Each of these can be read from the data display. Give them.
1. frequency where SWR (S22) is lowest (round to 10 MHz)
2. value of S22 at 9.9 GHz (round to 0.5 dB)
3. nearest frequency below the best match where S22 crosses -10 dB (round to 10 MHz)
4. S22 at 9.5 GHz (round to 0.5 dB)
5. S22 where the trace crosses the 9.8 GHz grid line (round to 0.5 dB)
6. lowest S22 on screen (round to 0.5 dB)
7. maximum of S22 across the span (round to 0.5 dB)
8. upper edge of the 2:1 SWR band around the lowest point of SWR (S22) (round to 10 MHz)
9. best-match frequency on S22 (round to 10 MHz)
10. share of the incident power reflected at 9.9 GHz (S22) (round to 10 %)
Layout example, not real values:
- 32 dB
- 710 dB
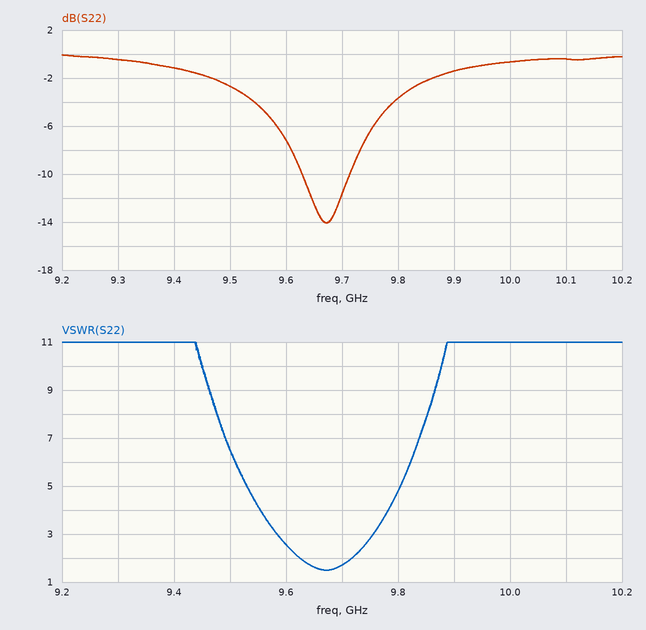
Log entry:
- 9.67 GHz
- -1.5 dB
- 9.63 GHz
- -2.5 dB
- -3.5 dB
- -14.0 dB
- 0.0 dB
- 9.72 GHz
- 9.67 GHz
- 70 %
